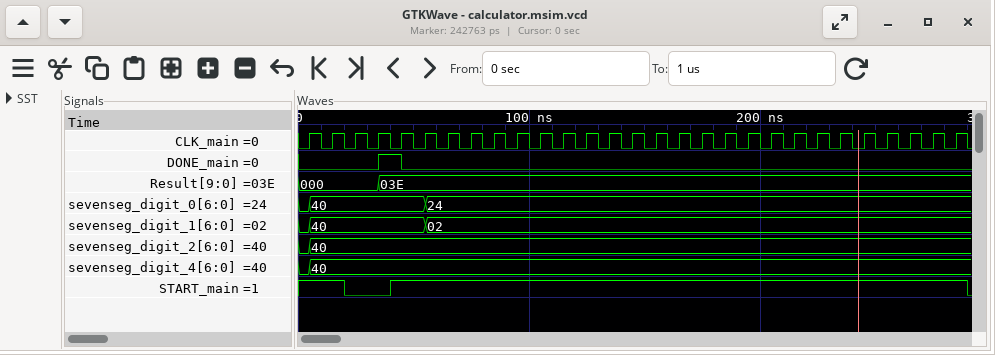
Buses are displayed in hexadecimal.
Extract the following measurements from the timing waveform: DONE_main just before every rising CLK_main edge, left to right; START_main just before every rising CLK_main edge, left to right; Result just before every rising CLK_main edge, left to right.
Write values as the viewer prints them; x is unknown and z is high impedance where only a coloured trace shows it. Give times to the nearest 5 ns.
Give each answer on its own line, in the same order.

0 0 0 0 1 0 0 0 0 0 0 0 0 0 0 0 0 0 0 0 0 0 0 0 0 0 0 0 0
1 1 0 0 1 1 1 1 1 1 1 1 1 1 1 1 1 1 1 1 1 1 1 1 1 1 1 1 1
000, 000, 000, 000, 03E, 03E, 03E, 03E, 03E, 03E, 03E, 03E, 03E, 03E, 03E, 03E, 03E, 03E, 03E, 03E, 03E, 03E, 03E, 03E, 03E, 03E, 03E, 03E, 03E
